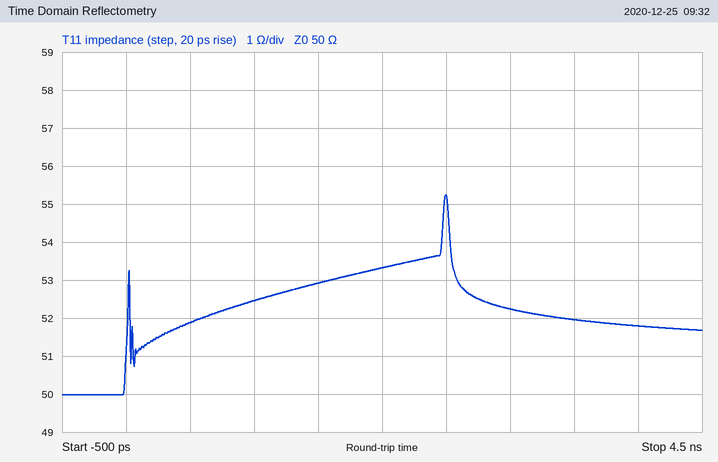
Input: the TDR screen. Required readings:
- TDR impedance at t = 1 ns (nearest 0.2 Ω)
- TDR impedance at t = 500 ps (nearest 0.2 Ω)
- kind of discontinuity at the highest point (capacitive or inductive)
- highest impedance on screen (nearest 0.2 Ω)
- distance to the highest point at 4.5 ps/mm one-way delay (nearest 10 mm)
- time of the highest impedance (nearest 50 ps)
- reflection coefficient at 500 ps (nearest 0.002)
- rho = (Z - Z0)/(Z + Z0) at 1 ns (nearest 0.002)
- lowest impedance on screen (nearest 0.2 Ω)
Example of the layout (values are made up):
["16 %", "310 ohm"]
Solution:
["52.4 Ω", "51.8 Ω", "inductive", "55.2 Ω", "280 mm", "2.50 ns", "+0.018", "+0.024", "50.0 Ω"]
